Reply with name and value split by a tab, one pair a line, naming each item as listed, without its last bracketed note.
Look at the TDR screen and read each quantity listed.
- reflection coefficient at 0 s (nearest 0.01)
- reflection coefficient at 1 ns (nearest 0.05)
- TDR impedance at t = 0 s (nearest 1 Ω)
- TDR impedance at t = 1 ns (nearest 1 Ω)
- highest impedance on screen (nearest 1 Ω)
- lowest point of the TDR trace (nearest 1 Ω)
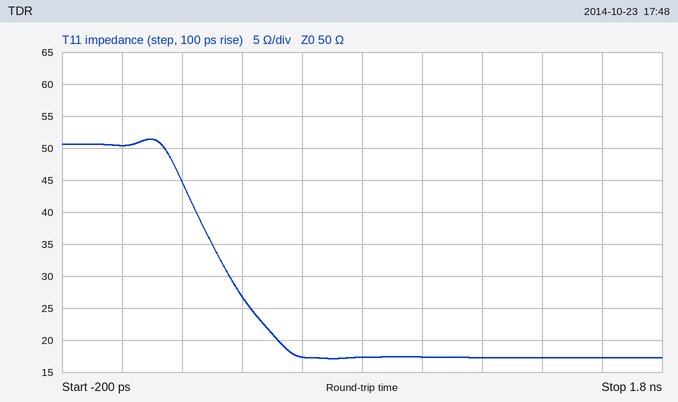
reflection coefficient at 0 s	0.00
reflection coefficient at 1 ns	-0.50
TDR impedance at t = 0 s	50 Ω
TDR impedance at t = 1 ns	17 Ω
highest impedance on screen	51 Ω
lowest point of the TDR trace	17 Ω
